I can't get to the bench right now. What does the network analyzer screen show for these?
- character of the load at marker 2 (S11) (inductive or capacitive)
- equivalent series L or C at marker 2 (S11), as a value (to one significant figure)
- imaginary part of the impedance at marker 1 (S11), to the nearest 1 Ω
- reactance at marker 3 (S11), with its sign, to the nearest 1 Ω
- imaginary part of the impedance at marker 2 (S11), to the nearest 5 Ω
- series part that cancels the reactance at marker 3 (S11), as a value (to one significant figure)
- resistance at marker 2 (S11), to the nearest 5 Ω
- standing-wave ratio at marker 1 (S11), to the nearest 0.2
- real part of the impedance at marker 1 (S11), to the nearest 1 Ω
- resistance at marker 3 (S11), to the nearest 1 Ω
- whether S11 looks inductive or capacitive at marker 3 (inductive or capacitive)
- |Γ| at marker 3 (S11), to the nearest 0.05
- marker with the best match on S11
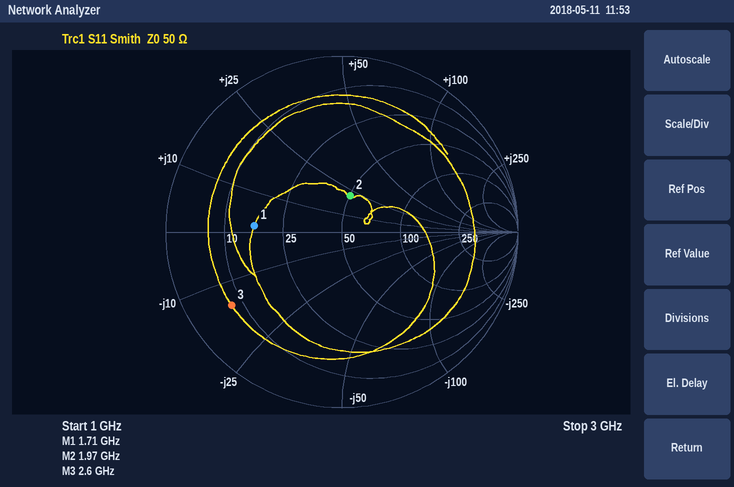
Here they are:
inductive
2 nH
+2 Ω
-15 Ω
+20 Ω
900 pH
50 Ω
3.0
17 Ω
8 Ω
capacitive
0.75
marker 2
